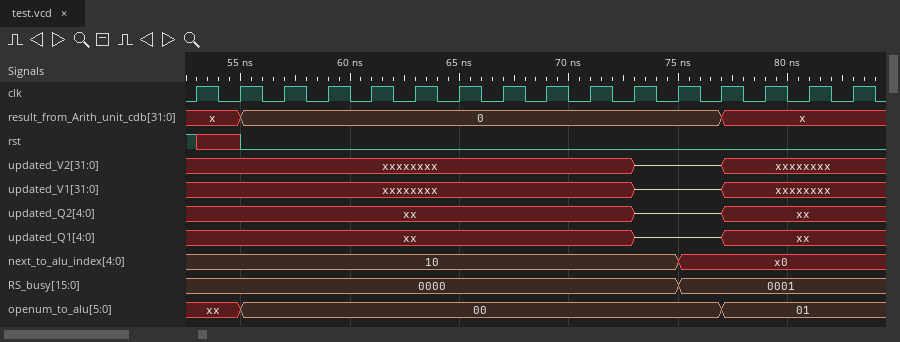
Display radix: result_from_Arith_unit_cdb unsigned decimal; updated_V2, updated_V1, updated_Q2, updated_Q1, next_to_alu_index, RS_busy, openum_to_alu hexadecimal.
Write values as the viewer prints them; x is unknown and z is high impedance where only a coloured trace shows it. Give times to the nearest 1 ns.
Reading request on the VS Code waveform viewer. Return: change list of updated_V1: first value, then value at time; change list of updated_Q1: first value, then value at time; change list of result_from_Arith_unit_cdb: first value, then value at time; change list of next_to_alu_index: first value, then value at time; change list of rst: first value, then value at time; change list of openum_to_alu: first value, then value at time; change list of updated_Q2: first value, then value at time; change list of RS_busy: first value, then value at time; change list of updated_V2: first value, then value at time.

xxxxxxxx, z at 73 ns, xxxxxxxx at 77 ns
xx, z at 73 ns, xx at 77 ns
x, 0 at 55 ns, x at 77 ns
10, x0 at 75 ns
1, x at 53 ns, 0 at 55 ns
xx, 00 at 55 ns, 01 at 77 ns
xx, z at 73 ns, xx at 77 ns
0000, 0001 at 75 ns
xxxxxxxx, z at 73 ns, xxxxxxxx at 77 ns
